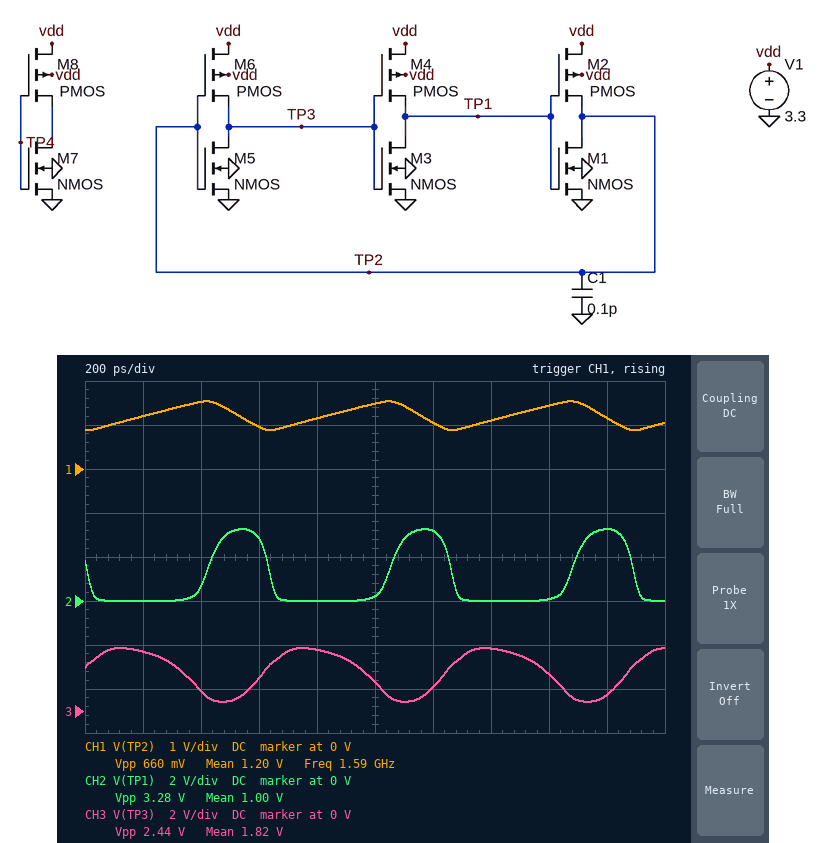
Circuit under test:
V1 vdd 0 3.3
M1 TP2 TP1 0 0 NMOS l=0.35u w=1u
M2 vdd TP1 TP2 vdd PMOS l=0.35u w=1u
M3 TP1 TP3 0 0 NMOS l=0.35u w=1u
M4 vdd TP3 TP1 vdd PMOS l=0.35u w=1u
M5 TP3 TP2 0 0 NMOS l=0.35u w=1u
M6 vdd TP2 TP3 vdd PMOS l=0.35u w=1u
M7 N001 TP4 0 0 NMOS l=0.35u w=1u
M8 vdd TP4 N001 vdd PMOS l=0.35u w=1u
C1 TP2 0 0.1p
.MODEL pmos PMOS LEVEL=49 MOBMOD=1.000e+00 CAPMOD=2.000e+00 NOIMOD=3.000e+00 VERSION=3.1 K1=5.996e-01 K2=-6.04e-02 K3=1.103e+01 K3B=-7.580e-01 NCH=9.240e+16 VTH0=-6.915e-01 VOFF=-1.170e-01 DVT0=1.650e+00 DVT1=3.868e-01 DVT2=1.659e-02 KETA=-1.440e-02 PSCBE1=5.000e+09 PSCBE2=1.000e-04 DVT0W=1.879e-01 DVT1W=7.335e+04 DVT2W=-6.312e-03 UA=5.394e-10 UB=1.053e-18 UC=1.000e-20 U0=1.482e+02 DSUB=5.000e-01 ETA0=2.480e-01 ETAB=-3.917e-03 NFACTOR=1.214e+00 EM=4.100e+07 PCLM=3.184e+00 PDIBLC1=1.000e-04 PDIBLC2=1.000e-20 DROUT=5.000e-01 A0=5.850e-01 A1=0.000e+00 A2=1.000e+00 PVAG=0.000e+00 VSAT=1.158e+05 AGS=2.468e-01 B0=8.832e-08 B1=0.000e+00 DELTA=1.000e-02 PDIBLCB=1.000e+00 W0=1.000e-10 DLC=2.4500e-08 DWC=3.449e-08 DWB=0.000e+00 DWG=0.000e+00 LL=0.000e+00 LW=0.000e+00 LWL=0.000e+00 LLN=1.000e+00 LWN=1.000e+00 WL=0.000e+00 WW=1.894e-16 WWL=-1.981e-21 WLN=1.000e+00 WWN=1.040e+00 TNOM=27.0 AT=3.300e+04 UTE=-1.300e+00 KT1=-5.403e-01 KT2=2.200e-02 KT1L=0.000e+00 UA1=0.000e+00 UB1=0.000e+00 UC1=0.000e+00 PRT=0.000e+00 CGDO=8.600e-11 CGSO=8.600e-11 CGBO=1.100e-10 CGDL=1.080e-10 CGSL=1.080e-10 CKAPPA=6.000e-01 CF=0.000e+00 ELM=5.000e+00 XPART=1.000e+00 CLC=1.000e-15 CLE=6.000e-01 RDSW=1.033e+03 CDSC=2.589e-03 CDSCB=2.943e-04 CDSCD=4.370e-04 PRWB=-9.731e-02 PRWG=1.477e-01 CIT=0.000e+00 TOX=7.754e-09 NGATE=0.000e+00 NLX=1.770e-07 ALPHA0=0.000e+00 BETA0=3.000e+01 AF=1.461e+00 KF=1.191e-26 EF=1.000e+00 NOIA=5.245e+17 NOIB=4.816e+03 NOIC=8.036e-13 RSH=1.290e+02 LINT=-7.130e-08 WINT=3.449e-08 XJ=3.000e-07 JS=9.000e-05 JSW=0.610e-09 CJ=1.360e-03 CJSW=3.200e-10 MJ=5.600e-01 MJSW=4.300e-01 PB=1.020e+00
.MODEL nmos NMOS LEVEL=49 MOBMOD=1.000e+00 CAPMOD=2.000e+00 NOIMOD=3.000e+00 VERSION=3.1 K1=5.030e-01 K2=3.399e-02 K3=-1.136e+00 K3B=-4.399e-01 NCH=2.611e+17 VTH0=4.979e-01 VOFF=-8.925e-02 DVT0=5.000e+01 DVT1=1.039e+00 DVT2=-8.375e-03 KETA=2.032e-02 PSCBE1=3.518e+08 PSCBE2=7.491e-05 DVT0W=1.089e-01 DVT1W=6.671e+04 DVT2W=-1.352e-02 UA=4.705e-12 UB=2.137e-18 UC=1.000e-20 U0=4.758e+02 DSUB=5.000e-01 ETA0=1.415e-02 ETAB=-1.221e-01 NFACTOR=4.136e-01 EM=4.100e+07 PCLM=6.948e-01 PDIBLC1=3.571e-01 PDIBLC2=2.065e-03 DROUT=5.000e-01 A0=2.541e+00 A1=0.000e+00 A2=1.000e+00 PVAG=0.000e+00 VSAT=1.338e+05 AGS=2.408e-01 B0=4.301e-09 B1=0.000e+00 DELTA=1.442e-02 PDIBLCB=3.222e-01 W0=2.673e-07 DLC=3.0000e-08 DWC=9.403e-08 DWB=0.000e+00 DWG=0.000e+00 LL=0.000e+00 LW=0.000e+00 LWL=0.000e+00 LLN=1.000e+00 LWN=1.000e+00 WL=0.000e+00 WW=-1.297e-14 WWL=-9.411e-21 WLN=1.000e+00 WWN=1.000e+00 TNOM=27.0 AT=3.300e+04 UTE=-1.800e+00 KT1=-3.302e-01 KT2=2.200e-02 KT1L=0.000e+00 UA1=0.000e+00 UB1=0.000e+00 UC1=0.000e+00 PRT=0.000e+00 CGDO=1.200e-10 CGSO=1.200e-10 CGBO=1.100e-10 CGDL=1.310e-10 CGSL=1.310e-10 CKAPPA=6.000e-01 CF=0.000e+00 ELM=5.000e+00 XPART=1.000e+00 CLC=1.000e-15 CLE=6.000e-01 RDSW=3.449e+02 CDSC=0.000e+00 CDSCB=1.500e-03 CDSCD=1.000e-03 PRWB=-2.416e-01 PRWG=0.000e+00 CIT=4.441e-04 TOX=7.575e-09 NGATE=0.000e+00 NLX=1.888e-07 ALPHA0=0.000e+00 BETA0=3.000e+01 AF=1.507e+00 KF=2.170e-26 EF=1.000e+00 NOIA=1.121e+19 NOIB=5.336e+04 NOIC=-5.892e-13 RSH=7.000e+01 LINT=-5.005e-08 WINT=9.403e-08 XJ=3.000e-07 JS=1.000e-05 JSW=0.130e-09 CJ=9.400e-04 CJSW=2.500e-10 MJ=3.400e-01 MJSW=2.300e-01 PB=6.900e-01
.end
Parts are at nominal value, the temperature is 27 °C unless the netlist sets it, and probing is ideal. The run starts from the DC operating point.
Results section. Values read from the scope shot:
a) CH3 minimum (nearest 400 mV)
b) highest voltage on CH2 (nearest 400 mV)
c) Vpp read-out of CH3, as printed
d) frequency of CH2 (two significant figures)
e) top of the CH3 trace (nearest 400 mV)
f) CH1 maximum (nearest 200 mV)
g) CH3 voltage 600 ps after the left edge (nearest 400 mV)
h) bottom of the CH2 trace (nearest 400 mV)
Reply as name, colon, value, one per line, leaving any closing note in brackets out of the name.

CH3 minimum: 400 mV
highest voltage on CH2: 3.2 V
Vpp read-out of CH3, as printed: 2.44 V
frequency of CH2: 1.6 GHz
top of the CH3 trace: 2.8 V
CH1 maximum: 1.6 V
CH3 voltage 600 ps after the left edge: 1.6 V
bottom of the CH2 trace: 0 V
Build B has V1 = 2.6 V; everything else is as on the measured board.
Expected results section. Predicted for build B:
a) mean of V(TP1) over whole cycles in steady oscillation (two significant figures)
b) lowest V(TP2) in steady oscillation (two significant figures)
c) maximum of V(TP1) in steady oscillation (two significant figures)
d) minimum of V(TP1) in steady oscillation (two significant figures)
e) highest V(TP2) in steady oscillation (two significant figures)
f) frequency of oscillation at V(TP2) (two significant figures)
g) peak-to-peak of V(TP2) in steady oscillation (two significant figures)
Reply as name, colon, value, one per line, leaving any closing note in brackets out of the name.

mean of V(TP1) over whole cycles in steady oscillation: 780 mV
lowest V(TP2) in steady oscillation: 670 mV
maximum of V(TP1) in steady oscillation: 2.6 V
minimum of V(TP1) in steady oscillation: -10 mV
highest V(TP2) in steady oscillation: 1.2 V
frequency of oscillation at V(TP2): 1.2 GHz
peak-to-peak of V(TP2) in steady oscillation: 570 mV
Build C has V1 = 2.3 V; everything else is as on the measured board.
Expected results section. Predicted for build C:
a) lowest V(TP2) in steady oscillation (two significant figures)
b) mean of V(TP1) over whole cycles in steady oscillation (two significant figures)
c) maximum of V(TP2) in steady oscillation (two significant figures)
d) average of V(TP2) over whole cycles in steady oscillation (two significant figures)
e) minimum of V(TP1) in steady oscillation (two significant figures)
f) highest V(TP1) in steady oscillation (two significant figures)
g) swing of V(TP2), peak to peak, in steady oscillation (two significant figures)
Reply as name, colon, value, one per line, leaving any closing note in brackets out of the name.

lowest V(TP2) in steady oscillation: 580 mV
mean of V(TP1) over whole cycles in steady oscillation: 680 mV
maximum of V(TP2) in steady oscillation: 1.1 V
average of V(TP2) over whole cycles in steady oscillation: 860 mV
minimum of V(TP1) in steady oscillation: -12 mV
highest V(TP1) in steady oscillation: 2.3 V
swing of V(TP2), peak to peak, in steady oscillation: 530 mV
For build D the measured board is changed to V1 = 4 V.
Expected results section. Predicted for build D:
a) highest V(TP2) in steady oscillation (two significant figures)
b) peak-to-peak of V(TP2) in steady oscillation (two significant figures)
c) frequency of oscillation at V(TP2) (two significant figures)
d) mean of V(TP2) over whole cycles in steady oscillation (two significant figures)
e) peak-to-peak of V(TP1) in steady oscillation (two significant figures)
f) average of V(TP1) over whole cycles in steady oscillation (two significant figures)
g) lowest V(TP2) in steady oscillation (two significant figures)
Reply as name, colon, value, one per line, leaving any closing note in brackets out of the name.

highest V(TP2) in steady oscillation: 1.8 V
peak-to-peak of V(TP2) in steady oscillation: 750 mV
frequency of oscillation at V(TP2): 1.9 GHz
mean of V(TP2) over whole cycles in steady oscillation: 1.5 V
peak-to-peak of V(TP1) in steady oscillation: 3.9 V
average of V(TP1) over whole cycles in steady oscillation: 1.3 V
lowest V(TP2) in steady oscillation: 1.1 V
